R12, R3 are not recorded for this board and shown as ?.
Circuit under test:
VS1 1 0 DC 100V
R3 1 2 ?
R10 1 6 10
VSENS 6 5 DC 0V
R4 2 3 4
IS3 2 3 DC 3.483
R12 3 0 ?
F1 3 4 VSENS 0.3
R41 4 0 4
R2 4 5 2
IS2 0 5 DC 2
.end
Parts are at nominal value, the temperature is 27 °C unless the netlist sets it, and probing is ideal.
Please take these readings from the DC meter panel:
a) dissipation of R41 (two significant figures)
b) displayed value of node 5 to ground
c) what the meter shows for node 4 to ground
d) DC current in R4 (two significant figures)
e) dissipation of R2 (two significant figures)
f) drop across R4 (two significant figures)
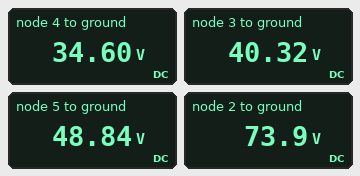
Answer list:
300 W
48.84 V
34.60 V
8.4 A
100 W
34 V
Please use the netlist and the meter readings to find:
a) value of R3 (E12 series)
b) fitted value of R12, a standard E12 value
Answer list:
2.2 Ω
3.9 Ω
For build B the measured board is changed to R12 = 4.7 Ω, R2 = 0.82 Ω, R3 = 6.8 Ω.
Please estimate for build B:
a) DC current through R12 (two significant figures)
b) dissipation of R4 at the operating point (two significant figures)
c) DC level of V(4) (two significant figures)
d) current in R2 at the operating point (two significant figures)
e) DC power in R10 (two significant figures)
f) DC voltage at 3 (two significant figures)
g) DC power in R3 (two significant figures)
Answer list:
6.2 A
77 W
37 V
7.6 A
320 W
29 V
420 W
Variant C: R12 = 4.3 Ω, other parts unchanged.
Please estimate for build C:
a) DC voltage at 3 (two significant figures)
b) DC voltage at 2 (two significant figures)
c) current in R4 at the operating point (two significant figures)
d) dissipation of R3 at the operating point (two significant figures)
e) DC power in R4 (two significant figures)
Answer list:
43 V
75 V
8.0 A
290 W
260 W
